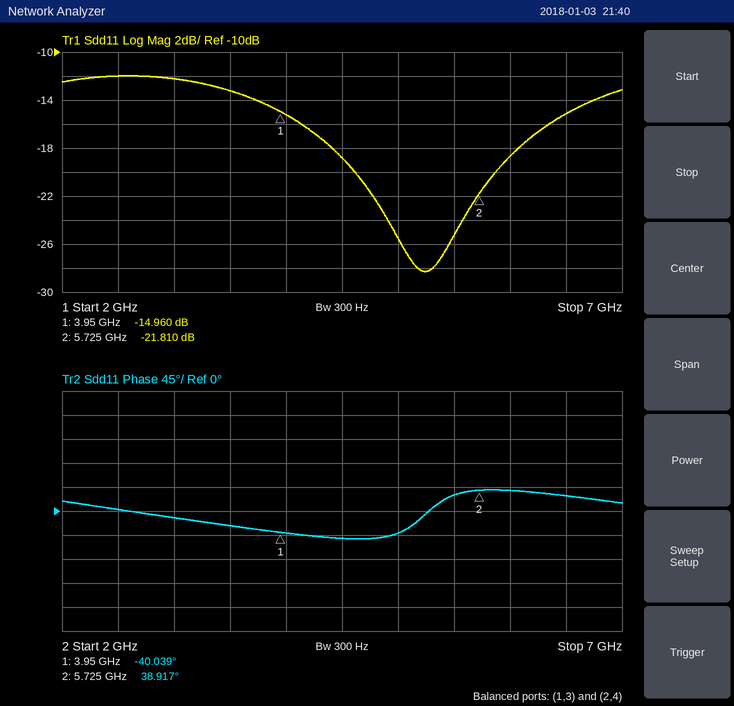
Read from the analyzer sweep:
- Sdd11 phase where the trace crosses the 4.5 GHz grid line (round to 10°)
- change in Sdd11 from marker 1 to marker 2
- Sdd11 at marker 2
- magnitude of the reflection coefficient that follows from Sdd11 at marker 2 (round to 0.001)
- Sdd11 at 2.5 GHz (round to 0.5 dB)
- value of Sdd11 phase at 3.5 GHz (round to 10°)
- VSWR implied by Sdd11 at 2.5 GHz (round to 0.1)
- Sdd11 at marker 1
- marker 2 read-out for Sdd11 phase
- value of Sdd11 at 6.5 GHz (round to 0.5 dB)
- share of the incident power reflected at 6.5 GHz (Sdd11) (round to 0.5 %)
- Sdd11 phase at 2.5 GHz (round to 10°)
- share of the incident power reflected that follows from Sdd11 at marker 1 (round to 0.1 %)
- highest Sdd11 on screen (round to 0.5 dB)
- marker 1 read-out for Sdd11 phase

-50°
-6.850 dB
-21.810 dB
0.081
-12.0 dB
-30°
1.7
-14.960 dB
38.917°
-15.0 dB
3.0 %
0°
3.2 %
-12.0 dB
-40.039°
